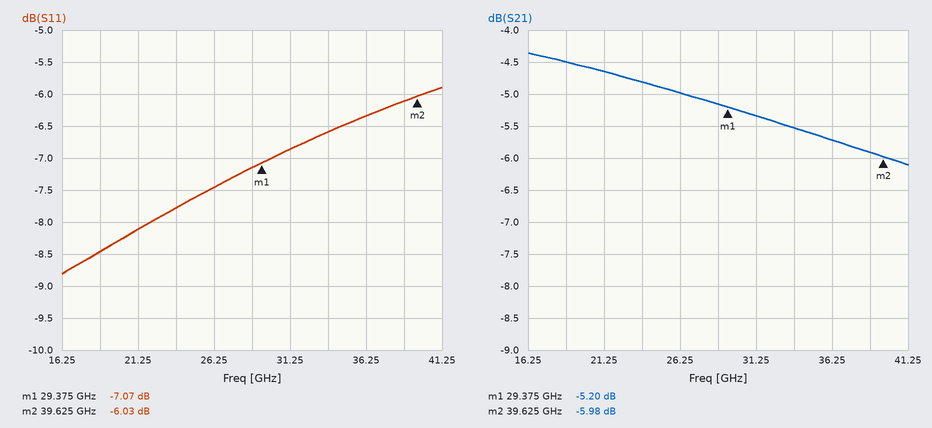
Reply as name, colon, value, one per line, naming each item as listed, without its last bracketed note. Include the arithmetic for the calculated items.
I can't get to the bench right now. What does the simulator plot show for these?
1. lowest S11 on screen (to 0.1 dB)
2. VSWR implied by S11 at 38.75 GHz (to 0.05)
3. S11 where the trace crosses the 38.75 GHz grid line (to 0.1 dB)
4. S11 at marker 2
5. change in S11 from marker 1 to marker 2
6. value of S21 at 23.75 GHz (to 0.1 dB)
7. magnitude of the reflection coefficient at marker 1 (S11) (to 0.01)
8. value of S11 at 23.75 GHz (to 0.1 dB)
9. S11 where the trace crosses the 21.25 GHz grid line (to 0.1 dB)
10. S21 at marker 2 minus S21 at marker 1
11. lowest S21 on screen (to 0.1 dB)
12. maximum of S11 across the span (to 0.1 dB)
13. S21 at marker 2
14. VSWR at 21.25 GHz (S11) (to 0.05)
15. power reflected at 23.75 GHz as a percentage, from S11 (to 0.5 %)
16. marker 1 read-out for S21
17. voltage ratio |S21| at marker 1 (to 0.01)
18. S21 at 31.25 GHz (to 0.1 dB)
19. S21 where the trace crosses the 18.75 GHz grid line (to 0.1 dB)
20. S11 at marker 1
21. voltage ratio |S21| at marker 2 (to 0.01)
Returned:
lowest S11 on screen: -8.8 dB
VSWR implied by S11 at 38.75 GHz: |Γ| = 10^(-6.1/20) = 0.4955; VSWR = (1 + 0.4955)/(1 − 0.4955) ≈ 2.96, so 2.95 to the nearest 0.05
S11 where the trace crosses the 38.75 GHz grid line: -6.1 dB
S11 at marker 2: -6.03 dB
change in S11 from marker 1 to marker 2: -6.03 − (-7.07) = 1.04 dB
value of S21 at 23.75 GHz: -4.8 dB
magnitude of the reflection coefficient at marker 1 (S11): 10^(-7.07/20) ≈ 0.44
value of S11 at 23.75 GHz: -7.8 dB
S11 where the trace crosses the 21.25 GHz grid line: -8.1 dB
S21 at marker 2 minus S21 at marker 1: -5.98 − (-5.2) = -0.78 dB
lowest S21 on screen: -6.1 dB
maximum of S11 across the span: -5.9 dB
S21 at marker 2: -5.98 dB
VSWR at 21.25 GHz (S11): |Γ| = 10^(-8.1/20) = 0.3936; VSWR = (1 + 0.3936)/(1 − 0.3936) ≈ 2.30
power reflected at 23.75 GHz as a percentage, from S11: 10^(-7.8/10) ≈ 16.6 %, so 16.5 % to the nearest 0.5 %
marker 1 read-out for S21: -5.20 dB
voltage ratio |S21| at marker 1: 10^(-5.2/20) ≈ 0.55
S21 at 31.25 GHz: -5.3 dB
S21 where the trace crosses the 18.75 GHz grid line: -4.5 dB
S11 at marker 1: -7.07 dB
voltage ratio |S21| at marker 2: 10^(-5.98/20) ≈ 0.50
